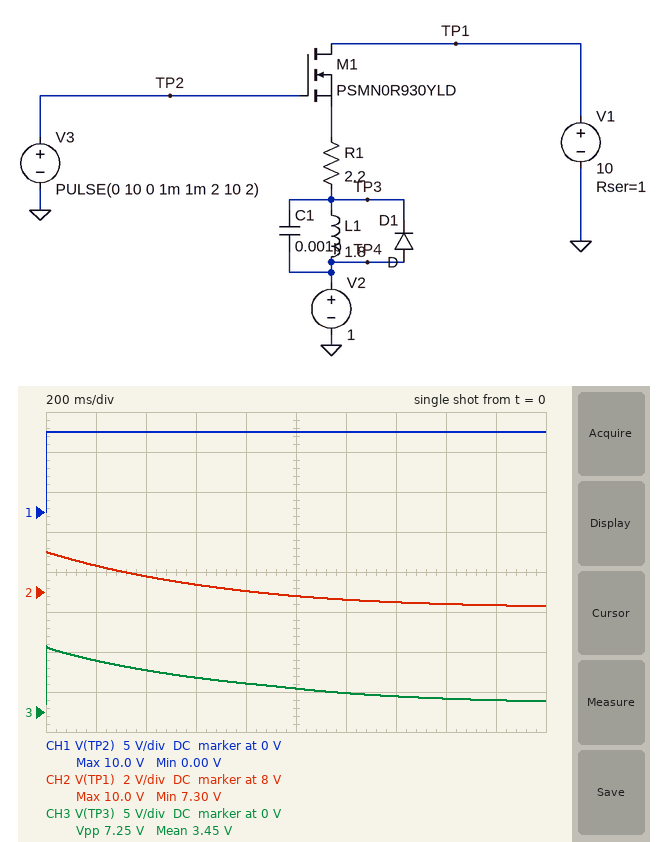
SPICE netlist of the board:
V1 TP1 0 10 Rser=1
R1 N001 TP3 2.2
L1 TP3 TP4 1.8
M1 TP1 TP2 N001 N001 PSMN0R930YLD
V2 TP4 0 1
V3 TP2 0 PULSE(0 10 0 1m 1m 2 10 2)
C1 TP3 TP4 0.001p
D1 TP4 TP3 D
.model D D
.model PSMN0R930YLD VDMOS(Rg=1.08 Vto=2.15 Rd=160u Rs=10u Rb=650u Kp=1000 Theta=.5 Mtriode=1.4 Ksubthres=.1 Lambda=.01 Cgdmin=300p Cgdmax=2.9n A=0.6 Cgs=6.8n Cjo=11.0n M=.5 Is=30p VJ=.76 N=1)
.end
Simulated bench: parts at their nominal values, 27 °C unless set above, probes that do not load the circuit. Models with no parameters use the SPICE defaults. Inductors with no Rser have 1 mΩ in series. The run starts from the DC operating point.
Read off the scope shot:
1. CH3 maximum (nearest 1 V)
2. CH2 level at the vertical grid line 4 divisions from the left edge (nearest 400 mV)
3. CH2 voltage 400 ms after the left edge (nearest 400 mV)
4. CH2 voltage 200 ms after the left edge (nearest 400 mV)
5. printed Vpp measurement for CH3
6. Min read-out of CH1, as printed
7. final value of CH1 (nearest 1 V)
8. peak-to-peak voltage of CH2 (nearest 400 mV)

8 V
8.0 V
8.8 V
9.2 V
7.25 V
0.00 V
10 V
2.8 V
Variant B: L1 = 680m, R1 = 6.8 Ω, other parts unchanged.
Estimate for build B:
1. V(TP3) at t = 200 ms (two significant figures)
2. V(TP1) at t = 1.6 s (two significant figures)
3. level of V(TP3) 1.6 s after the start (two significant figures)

1.9 V
9.0 V
1.0 V
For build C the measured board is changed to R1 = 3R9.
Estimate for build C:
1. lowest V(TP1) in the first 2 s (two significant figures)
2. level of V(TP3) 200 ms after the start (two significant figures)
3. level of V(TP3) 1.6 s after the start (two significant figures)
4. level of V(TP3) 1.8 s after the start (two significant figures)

8.3 V
5.5 V
1.2 V
1.1 V
